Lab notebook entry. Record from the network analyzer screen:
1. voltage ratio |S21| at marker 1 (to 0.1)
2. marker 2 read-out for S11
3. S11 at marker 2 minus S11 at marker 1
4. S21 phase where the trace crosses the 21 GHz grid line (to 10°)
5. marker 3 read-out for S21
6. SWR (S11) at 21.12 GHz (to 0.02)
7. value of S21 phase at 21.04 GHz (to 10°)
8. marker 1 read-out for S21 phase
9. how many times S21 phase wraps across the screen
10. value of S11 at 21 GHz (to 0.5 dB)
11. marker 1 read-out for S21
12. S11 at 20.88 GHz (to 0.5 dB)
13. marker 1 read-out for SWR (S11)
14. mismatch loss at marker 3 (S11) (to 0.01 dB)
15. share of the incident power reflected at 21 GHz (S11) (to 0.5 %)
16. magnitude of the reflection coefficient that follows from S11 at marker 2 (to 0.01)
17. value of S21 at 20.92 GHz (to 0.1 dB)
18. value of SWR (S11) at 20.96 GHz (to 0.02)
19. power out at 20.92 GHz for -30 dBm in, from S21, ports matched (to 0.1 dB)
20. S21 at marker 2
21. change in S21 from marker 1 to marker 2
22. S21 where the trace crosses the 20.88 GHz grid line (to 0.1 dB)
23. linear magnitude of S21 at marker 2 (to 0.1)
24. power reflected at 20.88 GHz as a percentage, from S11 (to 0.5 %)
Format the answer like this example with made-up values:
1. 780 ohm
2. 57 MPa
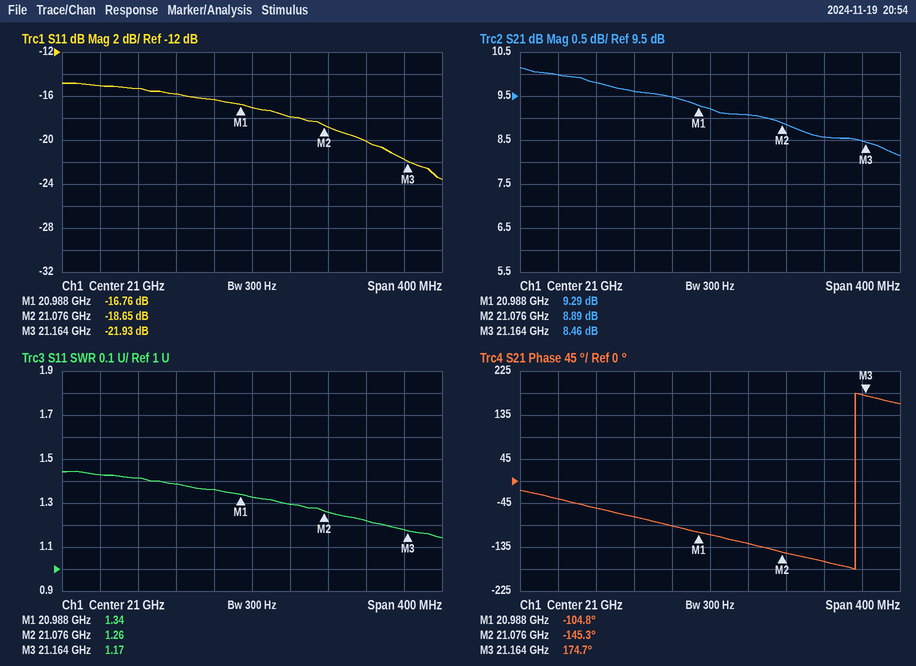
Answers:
1. 2.9
2. -18.65 dB
3. -1.89 dB
4. -110°
5. 8.46 dB
6. 1.22
7. -130°
8. -104.8°
9. 1
10. -17.0 dB
11. 9.29 dB
12. -15.5 dB
13. 1.34
14. 0.03 dB
15. 2.0 %
16. 0.12
17. 9.6 dB
18. 1.36
19. -20.4 dBm
20. 8.89 dB
21. -0.40 dB
22. 9.8 dB
23. 2.8
24. 3.0 %
